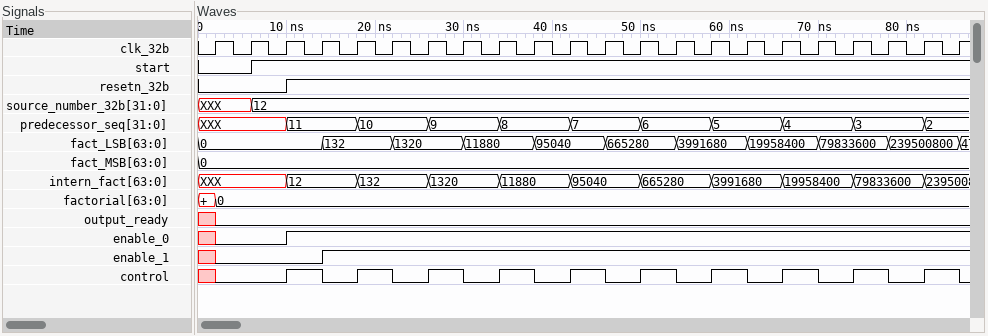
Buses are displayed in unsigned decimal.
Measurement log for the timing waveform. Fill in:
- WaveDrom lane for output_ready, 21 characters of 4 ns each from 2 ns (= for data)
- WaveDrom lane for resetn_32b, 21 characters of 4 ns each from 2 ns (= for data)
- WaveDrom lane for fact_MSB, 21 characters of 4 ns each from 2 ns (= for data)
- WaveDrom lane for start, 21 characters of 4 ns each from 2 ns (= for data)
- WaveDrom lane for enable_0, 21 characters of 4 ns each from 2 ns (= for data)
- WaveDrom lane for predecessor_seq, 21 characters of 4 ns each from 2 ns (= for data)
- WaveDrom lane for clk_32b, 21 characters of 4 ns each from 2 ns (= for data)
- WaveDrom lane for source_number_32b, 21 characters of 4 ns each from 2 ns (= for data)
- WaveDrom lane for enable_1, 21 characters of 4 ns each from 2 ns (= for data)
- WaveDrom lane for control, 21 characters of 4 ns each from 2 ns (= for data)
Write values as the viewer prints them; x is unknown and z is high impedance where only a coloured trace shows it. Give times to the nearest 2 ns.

{name: 'output_ready', wave: '0....................'}
{name: 'resetn_32b', wave: '0.1..................'}
{name: 'fact_MSB', wave: '=....................', data: '0'}
{name: 'start', wave: '01...................'}
{name: 'enable_0', wave: '0.1..................'}
{name: 'predecessor_seq', wave: 'x.=.=.=.=.=.=.=.=.=.=', data: '11 10 9 8 7 6 5 4 3 2'}
{name: 'clk_32b', wave: 'p....................'}
{name: 'source_number_32b', wave: 'x=...................', data: '12'}
{name: 'enable_1', wave: '0..1.................'}
{name: 'control', wave: '0.1010101010101010101'}
